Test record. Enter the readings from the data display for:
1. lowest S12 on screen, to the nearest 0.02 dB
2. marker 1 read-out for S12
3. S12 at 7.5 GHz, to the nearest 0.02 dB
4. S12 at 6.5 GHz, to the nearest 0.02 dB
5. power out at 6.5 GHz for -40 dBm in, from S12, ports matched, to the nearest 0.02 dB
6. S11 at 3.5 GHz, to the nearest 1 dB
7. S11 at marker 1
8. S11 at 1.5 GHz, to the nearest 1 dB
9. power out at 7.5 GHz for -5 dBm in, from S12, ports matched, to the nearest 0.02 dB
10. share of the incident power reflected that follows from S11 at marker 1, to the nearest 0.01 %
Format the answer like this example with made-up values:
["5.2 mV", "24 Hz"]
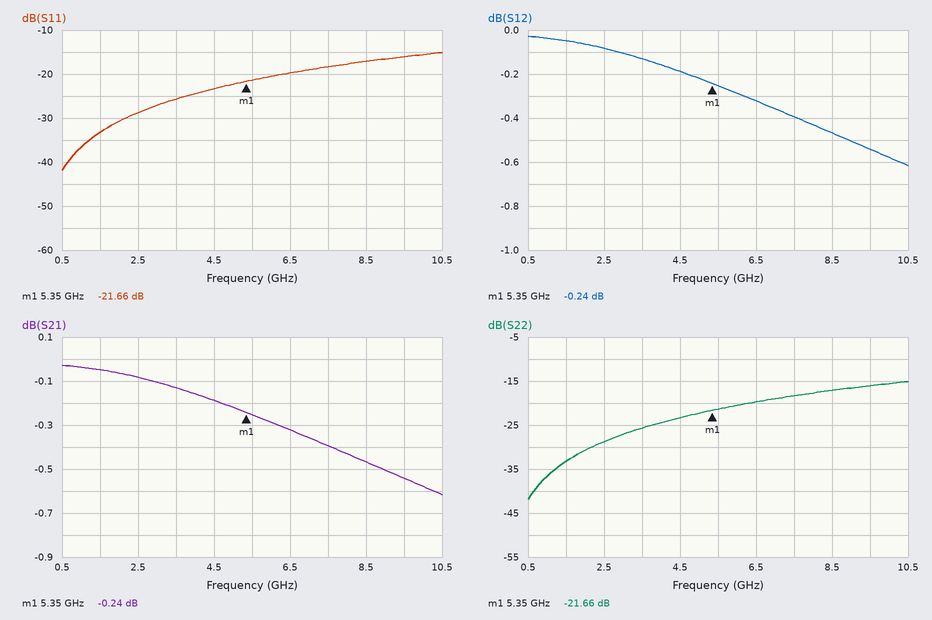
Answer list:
["-0.62 dB", "-0.24 dB", "-0.40 dB", "-0.32 dB", "-40.32 dBm", "-26 dB", "-21.66 dB", "-33 dB", "-5.40 dBm", "0.68 %"]
